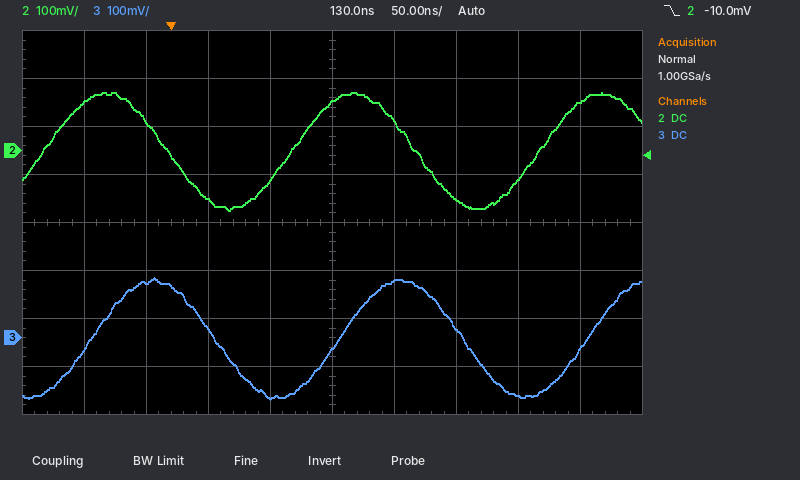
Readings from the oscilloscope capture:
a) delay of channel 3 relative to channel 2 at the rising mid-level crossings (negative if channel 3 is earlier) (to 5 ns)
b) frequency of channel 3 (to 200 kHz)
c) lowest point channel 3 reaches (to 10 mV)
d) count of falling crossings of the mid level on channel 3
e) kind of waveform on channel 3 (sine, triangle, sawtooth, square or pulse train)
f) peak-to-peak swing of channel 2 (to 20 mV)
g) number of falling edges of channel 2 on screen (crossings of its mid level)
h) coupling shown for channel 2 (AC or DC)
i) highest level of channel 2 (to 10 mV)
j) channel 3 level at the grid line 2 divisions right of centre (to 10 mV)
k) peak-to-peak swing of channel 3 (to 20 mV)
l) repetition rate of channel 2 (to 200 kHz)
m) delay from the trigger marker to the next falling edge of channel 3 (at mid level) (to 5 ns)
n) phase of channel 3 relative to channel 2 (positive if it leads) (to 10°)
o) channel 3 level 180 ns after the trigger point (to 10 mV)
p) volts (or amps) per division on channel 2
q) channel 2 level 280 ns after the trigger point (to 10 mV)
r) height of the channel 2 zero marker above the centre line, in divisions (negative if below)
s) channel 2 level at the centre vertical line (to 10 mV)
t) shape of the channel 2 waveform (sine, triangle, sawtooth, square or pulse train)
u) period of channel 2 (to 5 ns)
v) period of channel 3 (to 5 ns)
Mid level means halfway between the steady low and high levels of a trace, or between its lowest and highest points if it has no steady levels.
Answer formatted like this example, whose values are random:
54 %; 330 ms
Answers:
+40 ns; 5.0 MHz; -130 mV; 2; sine; 240 mV; 2; DC; 120 mV; 20 mV; 260 mV; 5.0 MHz; 35 ns; -70°; 120 mV; 100 mV; -60 mV; +1.5 div; 100 mV; sine; 200 ns; 200 ns
